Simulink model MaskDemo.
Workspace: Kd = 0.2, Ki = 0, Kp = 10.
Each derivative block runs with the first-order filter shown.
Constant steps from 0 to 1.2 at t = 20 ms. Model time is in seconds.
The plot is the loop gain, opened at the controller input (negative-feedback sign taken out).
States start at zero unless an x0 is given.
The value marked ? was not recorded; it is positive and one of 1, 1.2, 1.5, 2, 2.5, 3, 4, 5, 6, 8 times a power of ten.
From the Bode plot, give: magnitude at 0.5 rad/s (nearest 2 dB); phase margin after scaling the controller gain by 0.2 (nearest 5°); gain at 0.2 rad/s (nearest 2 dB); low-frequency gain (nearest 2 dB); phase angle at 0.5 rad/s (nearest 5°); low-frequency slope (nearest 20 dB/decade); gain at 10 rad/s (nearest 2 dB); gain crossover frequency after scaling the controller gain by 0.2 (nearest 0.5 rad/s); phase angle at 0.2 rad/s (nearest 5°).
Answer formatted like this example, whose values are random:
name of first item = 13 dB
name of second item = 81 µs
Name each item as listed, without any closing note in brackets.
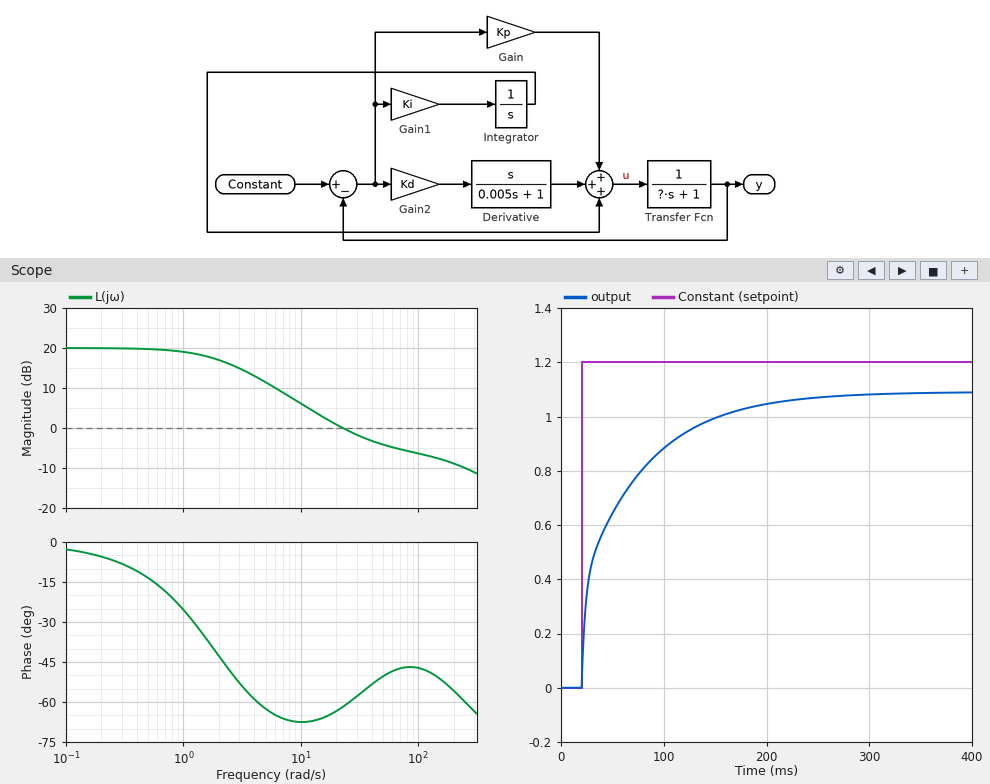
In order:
magnitude at 0.5 rad/s = 20 dB
phase margin after scaling the controller gain by 0.2 = 125°
gain at 0.2 rad/s = 20 dB
low-frequency gain = 20 dB
phase angle at 0.5 rad/s = -15°
low-frequency slope = 0 dB/decade
gain at 10 rad/s = 6 dB
gain crossover frequency after scaling the controller gain by 0.2 = 3.5 rad/s
phase angle at 0.2 rad/s = -5°
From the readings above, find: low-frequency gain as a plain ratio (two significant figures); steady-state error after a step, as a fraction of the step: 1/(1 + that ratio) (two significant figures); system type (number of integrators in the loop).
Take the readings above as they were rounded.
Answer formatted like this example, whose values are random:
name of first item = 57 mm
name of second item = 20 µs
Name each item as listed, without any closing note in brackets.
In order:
low-frequency gain as a plain ratio = 10
steady-state error after a step, as a fraction of the step: 1/(1 + that ratio) = 0.091
system type = 0
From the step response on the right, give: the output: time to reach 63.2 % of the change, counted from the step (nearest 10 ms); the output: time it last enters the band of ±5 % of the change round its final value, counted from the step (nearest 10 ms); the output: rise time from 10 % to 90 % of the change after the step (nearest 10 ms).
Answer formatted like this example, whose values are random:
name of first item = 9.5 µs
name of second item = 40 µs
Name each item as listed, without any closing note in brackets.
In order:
the output: time to reach 63.2 % of the change, counted from the step = 40 ms
the output: time it last enters the band of ±5 % of the change round its final value, counted from the step = 170 ms
the output: rise time from 10 % to 90 % of the change after the step = 120 ms
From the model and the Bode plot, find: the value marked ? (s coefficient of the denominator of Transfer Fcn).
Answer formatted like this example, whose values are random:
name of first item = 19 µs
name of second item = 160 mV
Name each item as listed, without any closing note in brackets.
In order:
the value marked ? = 0.5
